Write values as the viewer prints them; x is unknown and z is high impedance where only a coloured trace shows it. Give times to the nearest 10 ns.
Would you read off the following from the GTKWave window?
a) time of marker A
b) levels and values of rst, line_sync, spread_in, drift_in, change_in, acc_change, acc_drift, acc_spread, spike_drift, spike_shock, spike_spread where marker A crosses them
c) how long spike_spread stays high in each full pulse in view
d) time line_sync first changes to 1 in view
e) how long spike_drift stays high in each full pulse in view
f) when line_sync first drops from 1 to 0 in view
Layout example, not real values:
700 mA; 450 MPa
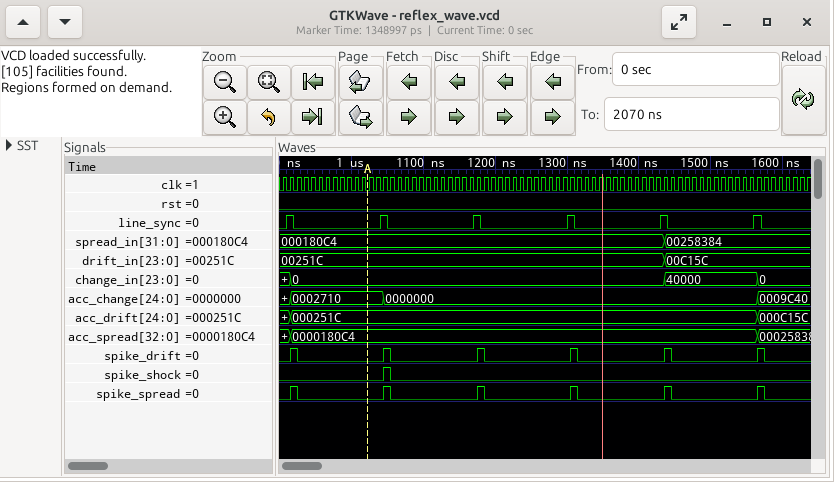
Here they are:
1020 ns; rst=0, line_sync=0, spread_in=000180C4, drift_in=00251C, change_in=0, acc_change=0002710, acc_drift=000251C, acc_spread=0000180C4, spike_drift=0, spike_shock=0, spike_spread=0; 10 ns, 10 ns, 10 ns, 10 ns, 10 ns, 10 ns; 910 ns; 10 ns, 10 ns, 10 ns, 10 ns, 10 ns, 10 ns; 920 ns
